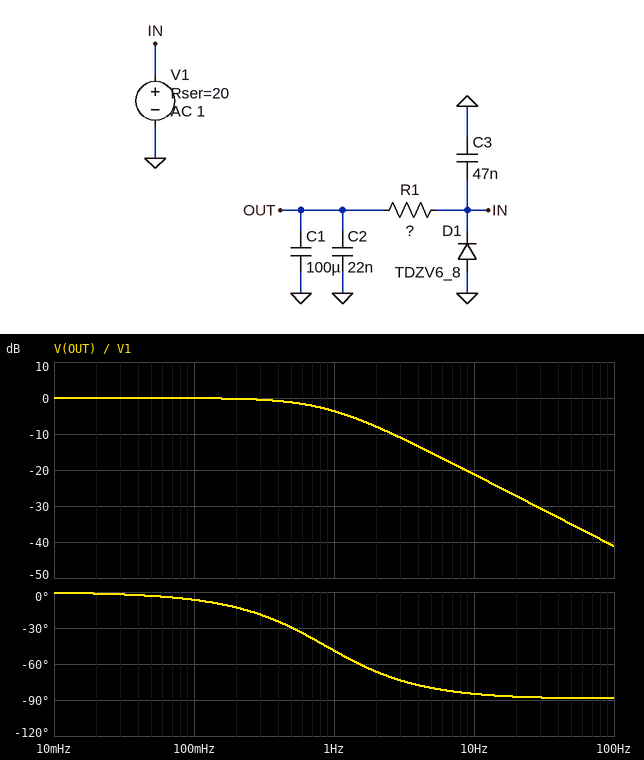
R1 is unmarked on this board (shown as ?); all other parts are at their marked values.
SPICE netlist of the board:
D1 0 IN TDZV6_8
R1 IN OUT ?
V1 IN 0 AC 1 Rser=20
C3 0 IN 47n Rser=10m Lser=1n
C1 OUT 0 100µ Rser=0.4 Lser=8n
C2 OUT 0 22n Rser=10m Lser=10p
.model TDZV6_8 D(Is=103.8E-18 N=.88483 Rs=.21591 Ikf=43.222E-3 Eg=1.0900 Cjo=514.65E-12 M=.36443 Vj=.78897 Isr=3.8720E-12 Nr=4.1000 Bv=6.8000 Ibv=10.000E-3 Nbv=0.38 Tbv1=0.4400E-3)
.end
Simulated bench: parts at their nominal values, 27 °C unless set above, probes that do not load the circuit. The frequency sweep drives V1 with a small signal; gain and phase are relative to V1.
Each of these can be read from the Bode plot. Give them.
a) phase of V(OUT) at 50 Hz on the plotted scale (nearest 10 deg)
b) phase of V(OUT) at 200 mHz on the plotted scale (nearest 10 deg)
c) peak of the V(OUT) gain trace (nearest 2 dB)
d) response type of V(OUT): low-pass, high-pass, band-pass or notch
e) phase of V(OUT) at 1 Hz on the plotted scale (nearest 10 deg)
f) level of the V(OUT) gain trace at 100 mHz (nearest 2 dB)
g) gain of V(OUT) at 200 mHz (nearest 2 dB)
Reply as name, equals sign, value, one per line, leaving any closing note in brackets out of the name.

phase of V(OUT) at 50 Hz on the plotted scale = -90 deg
phase of V(OUT) at 200 mHz on the plotted scale = -10 deg
peak of the V(OUT) gain trace = 0 dB
response type of V(OUT): low-pass, high-pass, band-pass or notch = low-pass
phase of V(OUT) at 1 Hz on the plotted scale = -50 deg
level of the V(OUT) gain trace at 100 mHz = 0 dB
gain of V(OUT) at 200 mHz = 0 dB
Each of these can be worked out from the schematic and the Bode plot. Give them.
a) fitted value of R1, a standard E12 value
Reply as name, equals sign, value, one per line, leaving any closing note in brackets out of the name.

fitted value of R1, a standard E12 value = 1.8 kΩ
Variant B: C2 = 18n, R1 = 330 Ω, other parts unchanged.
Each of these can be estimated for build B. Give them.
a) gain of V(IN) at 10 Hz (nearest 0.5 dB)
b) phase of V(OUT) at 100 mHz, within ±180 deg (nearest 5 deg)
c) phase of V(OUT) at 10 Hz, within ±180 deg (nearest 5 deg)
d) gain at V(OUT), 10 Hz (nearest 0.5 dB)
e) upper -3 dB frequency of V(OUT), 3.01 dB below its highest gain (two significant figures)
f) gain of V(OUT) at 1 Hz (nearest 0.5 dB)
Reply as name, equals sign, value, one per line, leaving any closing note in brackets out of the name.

gain of V(IN) at 10 Hz = -0.5 dB
phase of V(OUT) at 100 mHz, within ±180 deg = 0 deg
phase of V(OUT) at 10 Hz, within ±180 deg = -65 deg
gain at V(OUT), 10 Hz = -7.5 dB
upper -3 dB frequency of V(OUT), 3.01 dB below its highest gain = 4.5 Hz
gain of V(OUT) at 1 Hz = 0 dB
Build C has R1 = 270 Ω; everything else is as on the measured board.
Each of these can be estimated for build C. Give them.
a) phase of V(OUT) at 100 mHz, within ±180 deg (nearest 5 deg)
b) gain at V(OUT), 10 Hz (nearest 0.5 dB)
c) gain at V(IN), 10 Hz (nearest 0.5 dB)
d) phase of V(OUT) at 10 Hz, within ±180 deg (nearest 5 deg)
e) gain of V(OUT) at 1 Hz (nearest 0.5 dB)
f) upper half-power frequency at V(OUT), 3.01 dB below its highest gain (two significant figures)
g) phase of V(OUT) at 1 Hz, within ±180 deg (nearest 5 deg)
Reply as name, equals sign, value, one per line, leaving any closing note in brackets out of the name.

phase of V(OUT) at 100 mHz, within ±180 deg = 0 deg
gain at V(OUT), 10 Hz = -6.5 dB
gain at V(IN), 10 Hz = -0.5 dB
phase of V(OUT) at 10 Hz, within ±180 deg = -60 deg
gain of V(OUT) at 1 Hz = 0 dB
upper half-power frequency at V(OUT), 3.01 dB below its highest gain = 5.5 Hz
phase of V(OUT) at 1 Hz, within ±180 deg = -10 deg
